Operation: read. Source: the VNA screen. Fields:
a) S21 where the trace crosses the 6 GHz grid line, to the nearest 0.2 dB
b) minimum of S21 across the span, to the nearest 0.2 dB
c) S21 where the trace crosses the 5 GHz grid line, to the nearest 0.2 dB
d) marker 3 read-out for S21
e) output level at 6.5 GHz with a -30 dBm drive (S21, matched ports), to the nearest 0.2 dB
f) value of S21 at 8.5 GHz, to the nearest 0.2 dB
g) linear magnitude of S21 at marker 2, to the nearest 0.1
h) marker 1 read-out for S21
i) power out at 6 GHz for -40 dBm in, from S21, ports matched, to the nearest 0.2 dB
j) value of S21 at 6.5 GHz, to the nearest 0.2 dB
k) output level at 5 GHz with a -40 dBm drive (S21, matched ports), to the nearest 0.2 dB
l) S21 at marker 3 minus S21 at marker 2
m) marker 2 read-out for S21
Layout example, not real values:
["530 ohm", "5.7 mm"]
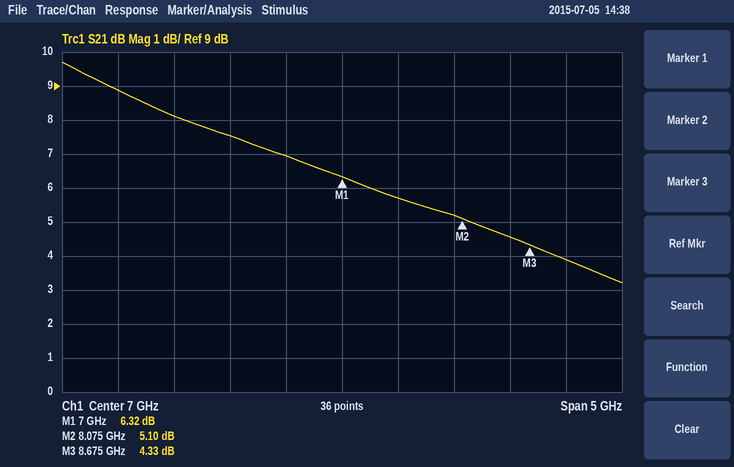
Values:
["7.6 dB", "3.2 dB", "8.8 dB", "4.33 dB", "-23.0 dBm", "4.6 dB", "1.8", "6.32 dB", "-32.4 dBm", "7.0 dB", "-31.2 dBm", "-0.77 dB", "5.10 dB"]
